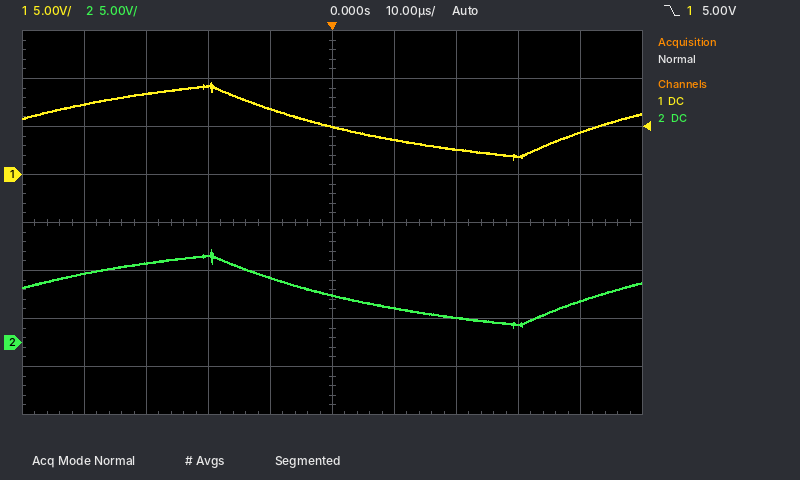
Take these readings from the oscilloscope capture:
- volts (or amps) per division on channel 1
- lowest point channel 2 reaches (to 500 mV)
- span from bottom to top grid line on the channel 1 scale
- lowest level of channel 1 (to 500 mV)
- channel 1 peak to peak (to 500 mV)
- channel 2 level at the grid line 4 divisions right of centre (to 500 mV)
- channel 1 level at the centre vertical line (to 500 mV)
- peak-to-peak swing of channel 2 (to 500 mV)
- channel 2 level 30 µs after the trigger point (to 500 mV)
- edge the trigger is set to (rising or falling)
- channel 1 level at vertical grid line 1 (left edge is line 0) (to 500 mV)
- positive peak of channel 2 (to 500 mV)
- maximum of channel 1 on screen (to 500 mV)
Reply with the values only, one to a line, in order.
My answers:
5 V
1.5 V
40 V
1.5 V
8.0 V
4.5 V
5.0 V
8.0 V
2.0 V
falling
7.5 V
9.5 V
9.5 V
